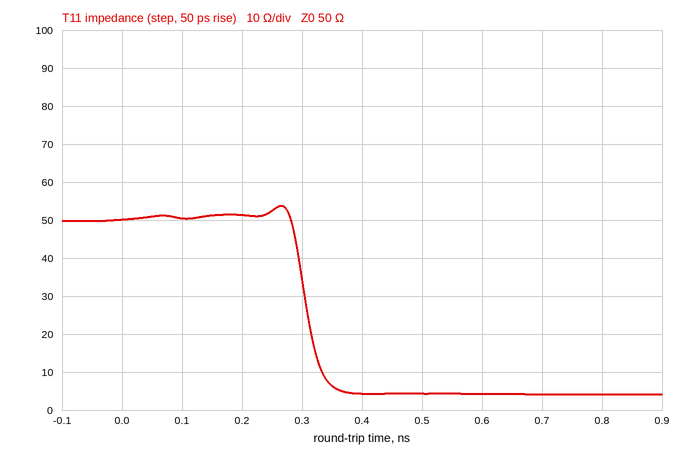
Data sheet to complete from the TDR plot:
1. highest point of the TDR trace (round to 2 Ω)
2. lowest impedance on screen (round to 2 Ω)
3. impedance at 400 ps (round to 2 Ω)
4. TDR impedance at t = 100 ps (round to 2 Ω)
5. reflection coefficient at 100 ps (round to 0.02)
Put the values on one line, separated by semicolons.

54 Ω; 4 Ω; 4 Ω; 50 Ω; 0.00
